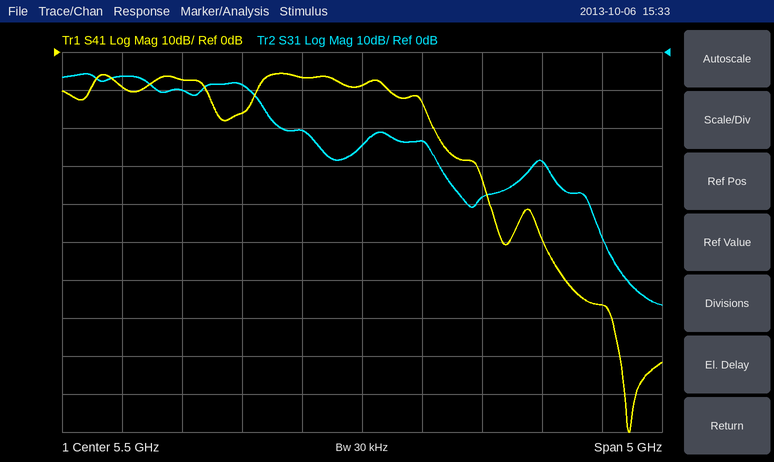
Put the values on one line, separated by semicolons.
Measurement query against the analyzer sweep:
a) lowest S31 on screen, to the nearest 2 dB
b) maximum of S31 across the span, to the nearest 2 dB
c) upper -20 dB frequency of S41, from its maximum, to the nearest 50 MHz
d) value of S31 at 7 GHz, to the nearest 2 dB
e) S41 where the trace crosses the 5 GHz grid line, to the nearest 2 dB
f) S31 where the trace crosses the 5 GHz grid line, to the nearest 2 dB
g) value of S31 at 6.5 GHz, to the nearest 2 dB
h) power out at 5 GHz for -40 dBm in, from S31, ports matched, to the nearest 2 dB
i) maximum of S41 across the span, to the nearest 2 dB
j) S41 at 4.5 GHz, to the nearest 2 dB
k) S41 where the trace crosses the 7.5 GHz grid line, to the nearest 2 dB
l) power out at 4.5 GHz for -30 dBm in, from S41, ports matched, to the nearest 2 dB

-66 dB; -6 dB; 6.20 GHz; -28 dB; -6 dB; -20 dB; -38 dB; -60 dBm; -6 dB; -16 dB; -66 dB; -46 dBm
